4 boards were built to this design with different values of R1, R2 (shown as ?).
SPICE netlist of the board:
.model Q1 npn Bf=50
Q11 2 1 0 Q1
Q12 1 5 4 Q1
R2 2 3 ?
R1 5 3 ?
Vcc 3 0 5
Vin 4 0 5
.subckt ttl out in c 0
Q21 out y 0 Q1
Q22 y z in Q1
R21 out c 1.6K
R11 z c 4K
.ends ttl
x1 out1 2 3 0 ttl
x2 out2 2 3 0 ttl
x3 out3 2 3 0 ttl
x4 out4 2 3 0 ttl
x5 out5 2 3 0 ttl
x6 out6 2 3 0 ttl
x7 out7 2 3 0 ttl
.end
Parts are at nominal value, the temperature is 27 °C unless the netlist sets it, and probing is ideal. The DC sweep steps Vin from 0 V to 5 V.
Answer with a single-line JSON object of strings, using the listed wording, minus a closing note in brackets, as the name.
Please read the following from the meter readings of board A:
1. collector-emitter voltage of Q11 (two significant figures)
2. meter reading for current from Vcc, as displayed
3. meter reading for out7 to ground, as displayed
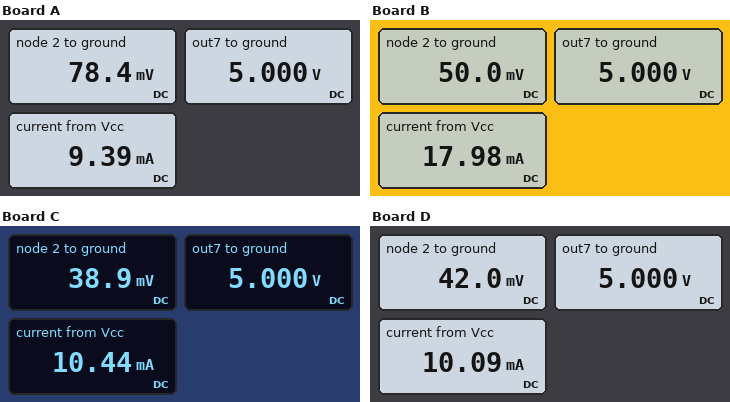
{"collector-emitter voltage of Q11": "78 mV", "meter reading for current from Vcc, as displayed": "9.39 mA", "meter reading for out7 to ground, as displayed": "5.000 V"}
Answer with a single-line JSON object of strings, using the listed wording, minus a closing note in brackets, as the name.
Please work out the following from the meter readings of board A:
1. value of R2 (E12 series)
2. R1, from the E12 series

{"value of R2": "2.7 kΩ", "R1, from the E12 series": "10 kΩ"}
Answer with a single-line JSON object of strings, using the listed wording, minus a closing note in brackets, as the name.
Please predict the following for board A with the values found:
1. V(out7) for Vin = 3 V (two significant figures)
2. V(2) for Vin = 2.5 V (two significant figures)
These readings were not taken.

{"V(out7) for Vin = 3 V": "5.0 V", "V(2) for Vin = 2.5 V": "78 mV"}
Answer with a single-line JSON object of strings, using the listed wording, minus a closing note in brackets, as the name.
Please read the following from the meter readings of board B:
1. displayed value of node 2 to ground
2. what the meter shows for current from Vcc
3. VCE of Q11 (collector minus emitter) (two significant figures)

{"displayed value of node 2 to ground": "50.0 mV", "what the meter shows for current from Vcc": "17.98 mA", "VCE of Q11 (collector minus emitter)": "50 mV"}
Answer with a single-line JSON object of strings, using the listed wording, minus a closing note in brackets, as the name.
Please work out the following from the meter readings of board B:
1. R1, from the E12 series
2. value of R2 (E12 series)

{"R1, from the E12 series": "1.8 kΩ", "value of R2": "560 Ω"}
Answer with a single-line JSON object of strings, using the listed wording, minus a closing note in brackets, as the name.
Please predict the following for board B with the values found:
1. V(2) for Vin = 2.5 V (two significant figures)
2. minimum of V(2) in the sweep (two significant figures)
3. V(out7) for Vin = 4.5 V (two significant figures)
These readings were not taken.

{"V(2) for Vin = 2.5 V": "50 mV", "minimum of V(2) in the sweep": "50 mV", "V(out7) for Vin = 4.5 V": "5.0 V"}
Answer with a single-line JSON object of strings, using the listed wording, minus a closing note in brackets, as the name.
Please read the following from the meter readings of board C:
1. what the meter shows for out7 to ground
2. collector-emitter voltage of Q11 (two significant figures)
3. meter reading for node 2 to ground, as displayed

{"what the meter shows for out7 to ground": "5.000 V", "collector-emitter voltage of Q11": "39 mV", "meter reading for node 2 to ground, as displayed": "38.9 mV"}
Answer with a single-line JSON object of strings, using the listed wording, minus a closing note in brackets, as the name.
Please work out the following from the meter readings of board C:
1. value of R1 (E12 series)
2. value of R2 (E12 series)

{"value of R1": "1.8 kΩ", "value of R2": "3.9 kΩ"}
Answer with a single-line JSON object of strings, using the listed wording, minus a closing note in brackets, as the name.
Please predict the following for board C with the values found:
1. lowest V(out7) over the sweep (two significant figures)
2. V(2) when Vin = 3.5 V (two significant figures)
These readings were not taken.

{"lowest V(out7) over the sweep": "44 mV", "V(2) when Vin = 3.5 V": "39 mV"}
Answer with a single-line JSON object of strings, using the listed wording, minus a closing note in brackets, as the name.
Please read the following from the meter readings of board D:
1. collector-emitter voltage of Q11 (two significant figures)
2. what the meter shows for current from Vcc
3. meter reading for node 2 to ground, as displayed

{"collector-emitter voltage of Q11": "42 mV", "what the meter shows for current from Vcc": "10.09 mA", "meter reading for node 2 to ground, as displayed": "42.0 mV"}
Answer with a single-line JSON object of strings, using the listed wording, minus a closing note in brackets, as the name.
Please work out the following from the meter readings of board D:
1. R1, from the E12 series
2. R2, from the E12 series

{"R1, from the E12 series": "2.2 kΩ", "R2, from the E12 series": "3.9 kΩ"}
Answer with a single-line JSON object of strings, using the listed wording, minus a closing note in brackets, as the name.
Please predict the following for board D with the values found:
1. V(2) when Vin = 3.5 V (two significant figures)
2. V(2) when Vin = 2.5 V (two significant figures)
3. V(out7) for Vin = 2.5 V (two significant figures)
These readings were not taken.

{"V(2) when Vin = 3.5 V": "42 mV", "V(2) when Vin = 2.5 V": "42 mV", "V(out7) for Vin = 2.5 V": "5.0 V"}
